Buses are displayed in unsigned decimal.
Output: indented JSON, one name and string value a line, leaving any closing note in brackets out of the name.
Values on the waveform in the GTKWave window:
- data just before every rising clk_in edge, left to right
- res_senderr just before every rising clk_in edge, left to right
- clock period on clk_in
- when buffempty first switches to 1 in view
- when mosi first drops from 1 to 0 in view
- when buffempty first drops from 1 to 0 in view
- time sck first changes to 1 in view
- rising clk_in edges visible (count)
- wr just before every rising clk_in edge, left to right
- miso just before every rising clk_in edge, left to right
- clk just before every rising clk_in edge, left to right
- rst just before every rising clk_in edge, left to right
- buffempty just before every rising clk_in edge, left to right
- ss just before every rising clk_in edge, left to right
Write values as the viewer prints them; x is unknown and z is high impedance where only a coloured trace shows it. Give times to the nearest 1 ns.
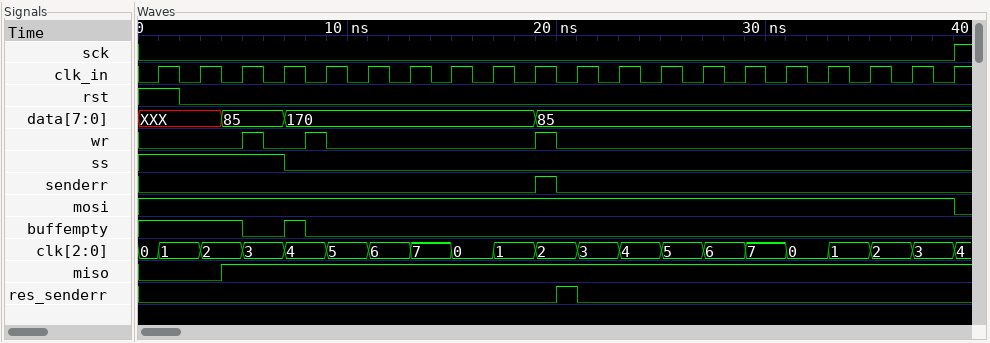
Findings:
{
  "data just before every rising clk_in edge, left to right": "XXX, XXX, 85, 85, 170, 170, 170, 170, 170, 170, 85, 85, 85, 85, 85, 85, 85, 85, 85, 85",
  "res_senderr just before every rising clk_in edge, left to right": "0 0 0 0 0 0 0 0 0 0 1 0 0 0 0 0 0 0 0 0",
  "clock period on clk_in": "2 ns",
  "when buffempty first switches to 1 in view": "7 ns",
  "when mosi first drops from 1 to 0 in view": "39 ns",
  "when buffempty first drops from 1 to 0 in view": "5 ns",
  "time sck first changes to 1 in view": "39 ns",
  "rising clk_in edges visible": "20",
  "wr just before every rising clk_in edge, left to right": "0 0 0 0 1 0 0 0 0 0 0 0 0 0 0 0 0 0 0 0",
  "miso just before every rising clk_in edge, left to right": "0 0 1 1 1 1 1 1 1 1 1 1 1 1 1 1 1 1 1 1",
  "clk just before every rising clk_in edge, left to right": "0, 1, 2, 3, 4, 5, 6, 7, 0, 1, 2, 3, 4, 5, 6, 7, 0, 1, 2, 3",
  "rst just before every rising clk_in edge, left to right": "1 0 0 0 0 0 0 0 0 0 0 0 0 0 0 0 0 0 0 0",
  "buffempty just before every rising clk_in edge, left to right": "1 1 1 0 0 0 0 0 0 0 0 0 0 0 0 0 0 0 0 0",
  "ss just before every rising clk_in edge, left to right": "1 1 1 1 0 0 0 0 0 0 0 0 0 0 0 0 0 0 0 0"
}
